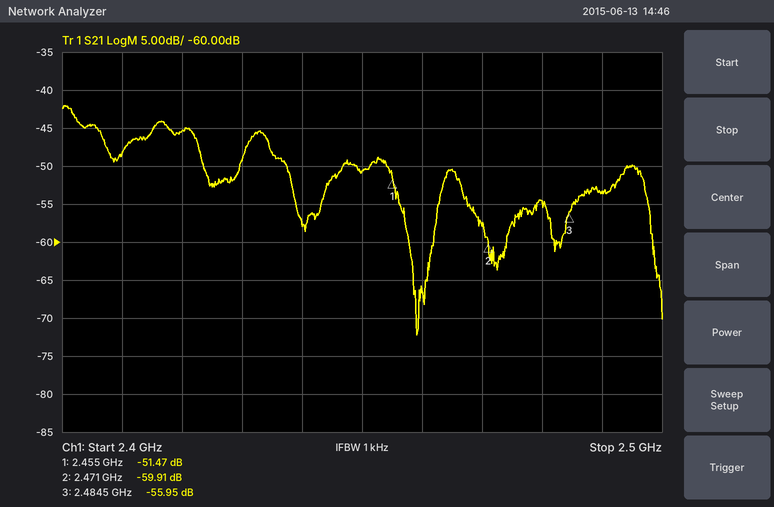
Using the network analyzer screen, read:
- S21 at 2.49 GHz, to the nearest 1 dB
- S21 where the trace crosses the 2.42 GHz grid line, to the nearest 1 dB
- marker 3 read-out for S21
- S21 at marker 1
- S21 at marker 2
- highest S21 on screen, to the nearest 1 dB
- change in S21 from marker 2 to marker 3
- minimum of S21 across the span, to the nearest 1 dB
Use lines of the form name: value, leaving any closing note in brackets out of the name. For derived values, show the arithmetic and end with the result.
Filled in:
S21 at 2.49 GHz, to the nearest 1 dB: -53 dB
S21 where the trace crosses the 2.42 GHz grid line, to the nearest 1 dB: -45 dB
marker 3 read-out for S21: -55.95 dB
S21 at marker 1: -51.47 dB
S21 at marker 2: -59.91 dB
highest S21 on screen, to the nearest 1 dB: -42 dB
change in S21 from marker 2 to marker 3: -55.95 − (-59.91) = 3.96 dB
minimum of S21 across the span, to the nearest 1 dB: -72 dB
